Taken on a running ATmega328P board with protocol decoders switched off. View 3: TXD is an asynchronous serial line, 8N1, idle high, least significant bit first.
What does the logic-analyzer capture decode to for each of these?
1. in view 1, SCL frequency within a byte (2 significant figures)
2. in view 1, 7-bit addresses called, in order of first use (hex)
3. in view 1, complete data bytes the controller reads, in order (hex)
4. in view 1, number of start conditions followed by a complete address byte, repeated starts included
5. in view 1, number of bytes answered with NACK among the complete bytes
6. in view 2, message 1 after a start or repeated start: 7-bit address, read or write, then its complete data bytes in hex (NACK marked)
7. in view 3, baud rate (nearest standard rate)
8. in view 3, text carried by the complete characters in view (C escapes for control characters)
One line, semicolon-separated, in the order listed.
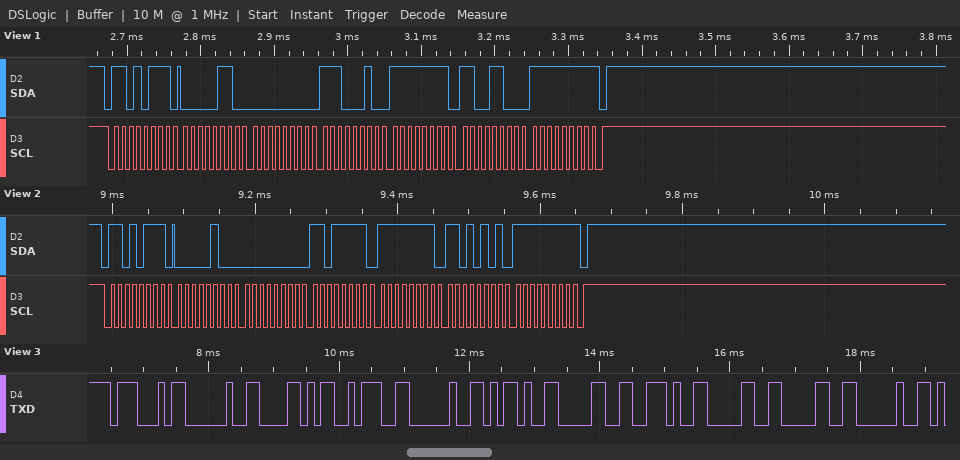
100 kHz; 0x6B; 06 00 E2 FF CC FF; 1; 1; 0x6B read: 04 00 DF FF D5 FF NACK; 9600 baud; "G X: -0.00 "
